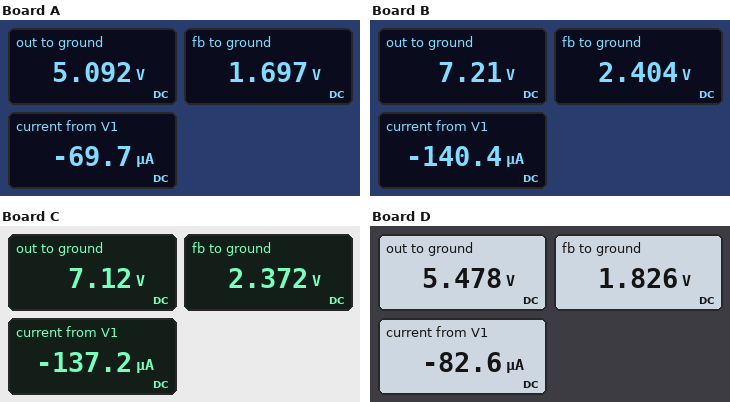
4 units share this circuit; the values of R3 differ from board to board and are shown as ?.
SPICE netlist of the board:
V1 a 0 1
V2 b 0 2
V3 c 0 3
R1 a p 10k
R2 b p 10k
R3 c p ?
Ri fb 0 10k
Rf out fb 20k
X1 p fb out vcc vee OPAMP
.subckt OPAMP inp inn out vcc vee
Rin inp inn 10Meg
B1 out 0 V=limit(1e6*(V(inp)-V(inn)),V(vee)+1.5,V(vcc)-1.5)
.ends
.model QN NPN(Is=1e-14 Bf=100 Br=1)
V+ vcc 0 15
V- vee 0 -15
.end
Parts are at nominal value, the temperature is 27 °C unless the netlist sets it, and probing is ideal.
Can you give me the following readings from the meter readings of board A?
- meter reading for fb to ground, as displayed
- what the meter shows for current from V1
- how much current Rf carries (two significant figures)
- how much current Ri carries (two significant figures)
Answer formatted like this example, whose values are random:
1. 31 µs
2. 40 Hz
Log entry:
1. 1.697 V
2. -69.7 µA
3. 170 µA
4. 170 µA
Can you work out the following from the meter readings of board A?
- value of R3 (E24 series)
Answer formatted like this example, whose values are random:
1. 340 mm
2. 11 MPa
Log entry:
1. 33 kΩ
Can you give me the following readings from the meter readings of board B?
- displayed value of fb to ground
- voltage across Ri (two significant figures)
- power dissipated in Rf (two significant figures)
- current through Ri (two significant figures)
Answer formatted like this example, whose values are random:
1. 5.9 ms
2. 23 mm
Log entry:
1. 2.404 V
2. 2.4 V
3. 1.2 mW
4. 240 µA
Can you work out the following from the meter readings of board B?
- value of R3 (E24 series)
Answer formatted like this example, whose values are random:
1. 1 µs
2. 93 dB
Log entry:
1. 3.3 kΩ
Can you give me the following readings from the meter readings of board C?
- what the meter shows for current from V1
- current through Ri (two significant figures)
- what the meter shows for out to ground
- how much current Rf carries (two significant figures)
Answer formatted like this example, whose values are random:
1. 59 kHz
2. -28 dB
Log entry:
1. -137.2 µA
2. 240 µA
3. 7.12 V
4. 240 µA
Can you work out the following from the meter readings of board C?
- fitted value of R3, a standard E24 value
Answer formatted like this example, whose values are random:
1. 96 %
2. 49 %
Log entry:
1. 3.6 kΩ
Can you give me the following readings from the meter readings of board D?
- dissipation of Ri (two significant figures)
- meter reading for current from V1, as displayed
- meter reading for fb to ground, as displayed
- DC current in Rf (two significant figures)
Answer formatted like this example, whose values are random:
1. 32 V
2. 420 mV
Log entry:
1. 330 µW
2. -82.6 µA
3. 1.826 V
4. 180 µA
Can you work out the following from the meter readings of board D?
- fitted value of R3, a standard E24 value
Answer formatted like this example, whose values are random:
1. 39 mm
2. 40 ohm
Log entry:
1. 18 kΩ
